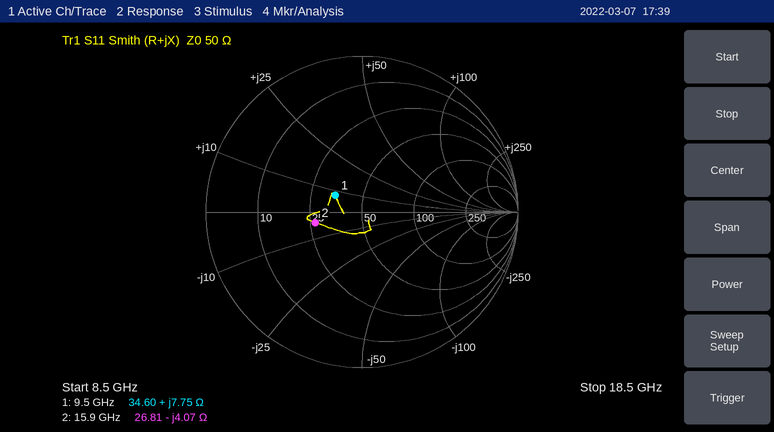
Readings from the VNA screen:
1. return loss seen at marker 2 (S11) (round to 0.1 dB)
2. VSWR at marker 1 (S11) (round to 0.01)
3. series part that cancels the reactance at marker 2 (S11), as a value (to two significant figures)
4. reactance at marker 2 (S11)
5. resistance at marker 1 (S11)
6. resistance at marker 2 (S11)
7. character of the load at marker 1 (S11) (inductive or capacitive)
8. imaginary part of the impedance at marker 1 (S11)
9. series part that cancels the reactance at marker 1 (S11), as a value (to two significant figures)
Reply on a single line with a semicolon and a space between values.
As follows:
10.3 dB; 1.51; 41 pH; -4.07 Ω; 34.60 Ω; 26.81 Ω; inductive; +7.75 Ω; 2.2 pF
